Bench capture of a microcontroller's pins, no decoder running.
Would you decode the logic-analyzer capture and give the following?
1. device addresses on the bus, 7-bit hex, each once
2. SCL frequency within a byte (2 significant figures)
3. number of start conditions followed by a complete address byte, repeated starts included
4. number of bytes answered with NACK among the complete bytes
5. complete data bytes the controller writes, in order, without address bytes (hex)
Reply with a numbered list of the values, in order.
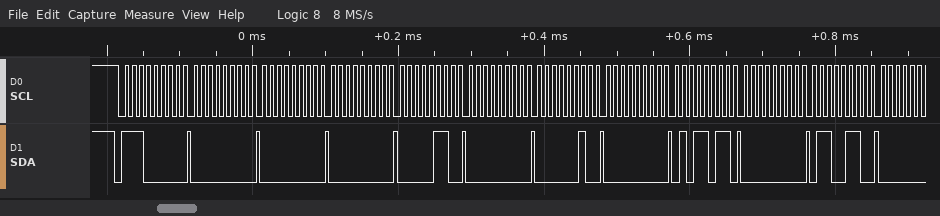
1. 0x70
2. 100 kHz
3. 1
4. 0
5. 00 00 00 06 00 02 00 5B 00 66
